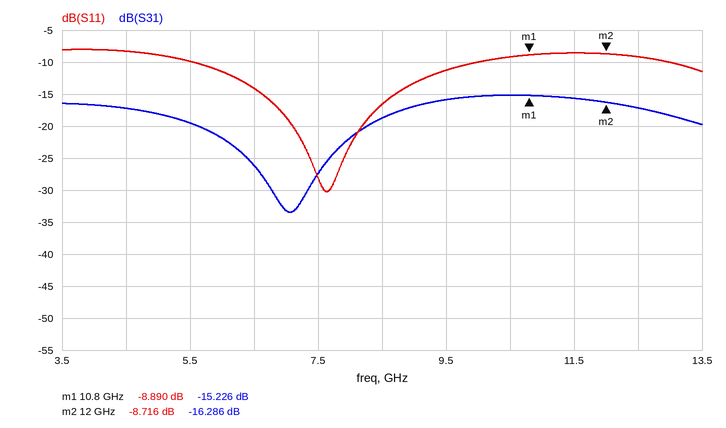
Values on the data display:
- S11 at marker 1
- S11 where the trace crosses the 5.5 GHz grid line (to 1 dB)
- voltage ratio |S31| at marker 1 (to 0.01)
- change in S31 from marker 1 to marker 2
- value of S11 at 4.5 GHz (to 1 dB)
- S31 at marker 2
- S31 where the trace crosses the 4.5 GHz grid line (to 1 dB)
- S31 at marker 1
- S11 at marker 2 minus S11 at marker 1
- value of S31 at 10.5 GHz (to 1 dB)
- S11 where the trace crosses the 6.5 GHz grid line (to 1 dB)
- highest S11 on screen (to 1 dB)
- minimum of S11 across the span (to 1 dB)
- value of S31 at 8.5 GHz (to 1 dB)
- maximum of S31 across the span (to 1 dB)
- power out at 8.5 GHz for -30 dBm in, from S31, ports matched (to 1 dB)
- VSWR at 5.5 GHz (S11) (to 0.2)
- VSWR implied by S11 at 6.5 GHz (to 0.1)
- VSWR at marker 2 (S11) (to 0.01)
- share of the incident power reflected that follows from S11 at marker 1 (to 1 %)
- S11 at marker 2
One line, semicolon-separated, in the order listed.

-8.890 dB; -10 dB; 0.17; -1.060 dB; -8 dB; -16.286 dB; -17 dB; -15.226 dB; 0.174 dB; -15 dB; -14 dB; -8 dB; -30 dB; -19 dB; -15 dB; -49 dBm; 2.0; 1.5; 2.16; 13 %; -8.716 dB
